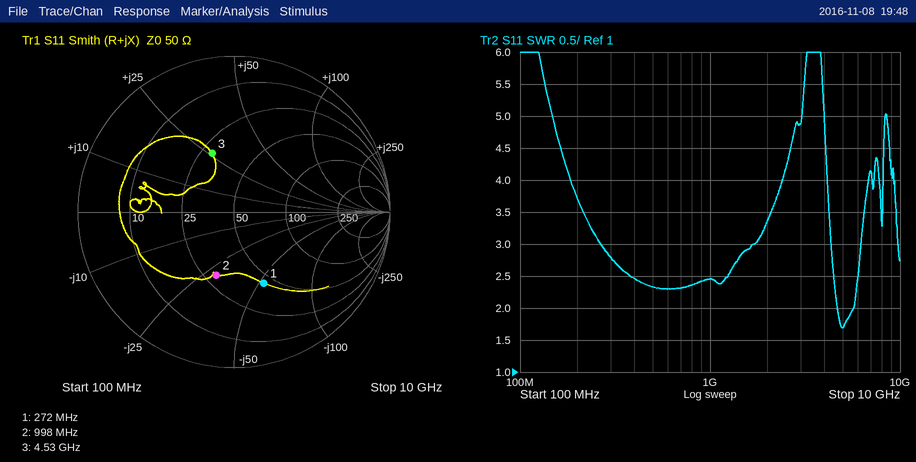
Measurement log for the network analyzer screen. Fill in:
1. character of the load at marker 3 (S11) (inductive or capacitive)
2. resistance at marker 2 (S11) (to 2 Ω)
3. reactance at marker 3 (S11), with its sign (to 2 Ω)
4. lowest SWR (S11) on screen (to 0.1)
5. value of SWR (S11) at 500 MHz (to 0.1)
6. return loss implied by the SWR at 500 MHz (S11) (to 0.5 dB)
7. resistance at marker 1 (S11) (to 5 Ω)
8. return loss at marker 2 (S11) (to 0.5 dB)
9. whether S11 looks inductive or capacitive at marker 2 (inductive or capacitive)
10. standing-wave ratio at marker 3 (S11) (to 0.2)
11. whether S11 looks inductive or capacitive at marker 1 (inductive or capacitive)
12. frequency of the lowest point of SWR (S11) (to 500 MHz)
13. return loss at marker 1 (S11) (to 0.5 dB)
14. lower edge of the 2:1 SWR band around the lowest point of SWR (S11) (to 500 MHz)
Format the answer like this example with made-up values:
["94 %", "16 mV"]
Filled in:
["inductive", "30 Ω", "+26 Ω", "1.7", "2.3", "8.0 dB", "45 Ω", "7.5 dB", "capacitive", "2.4", "capacitive", "5.0 GHz", "6.0 dB", "4.5 GHz"]
